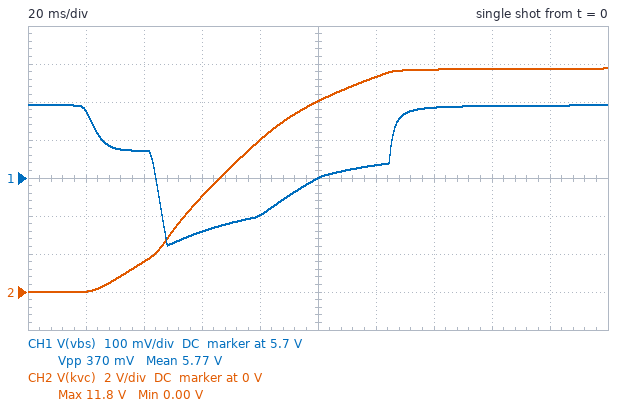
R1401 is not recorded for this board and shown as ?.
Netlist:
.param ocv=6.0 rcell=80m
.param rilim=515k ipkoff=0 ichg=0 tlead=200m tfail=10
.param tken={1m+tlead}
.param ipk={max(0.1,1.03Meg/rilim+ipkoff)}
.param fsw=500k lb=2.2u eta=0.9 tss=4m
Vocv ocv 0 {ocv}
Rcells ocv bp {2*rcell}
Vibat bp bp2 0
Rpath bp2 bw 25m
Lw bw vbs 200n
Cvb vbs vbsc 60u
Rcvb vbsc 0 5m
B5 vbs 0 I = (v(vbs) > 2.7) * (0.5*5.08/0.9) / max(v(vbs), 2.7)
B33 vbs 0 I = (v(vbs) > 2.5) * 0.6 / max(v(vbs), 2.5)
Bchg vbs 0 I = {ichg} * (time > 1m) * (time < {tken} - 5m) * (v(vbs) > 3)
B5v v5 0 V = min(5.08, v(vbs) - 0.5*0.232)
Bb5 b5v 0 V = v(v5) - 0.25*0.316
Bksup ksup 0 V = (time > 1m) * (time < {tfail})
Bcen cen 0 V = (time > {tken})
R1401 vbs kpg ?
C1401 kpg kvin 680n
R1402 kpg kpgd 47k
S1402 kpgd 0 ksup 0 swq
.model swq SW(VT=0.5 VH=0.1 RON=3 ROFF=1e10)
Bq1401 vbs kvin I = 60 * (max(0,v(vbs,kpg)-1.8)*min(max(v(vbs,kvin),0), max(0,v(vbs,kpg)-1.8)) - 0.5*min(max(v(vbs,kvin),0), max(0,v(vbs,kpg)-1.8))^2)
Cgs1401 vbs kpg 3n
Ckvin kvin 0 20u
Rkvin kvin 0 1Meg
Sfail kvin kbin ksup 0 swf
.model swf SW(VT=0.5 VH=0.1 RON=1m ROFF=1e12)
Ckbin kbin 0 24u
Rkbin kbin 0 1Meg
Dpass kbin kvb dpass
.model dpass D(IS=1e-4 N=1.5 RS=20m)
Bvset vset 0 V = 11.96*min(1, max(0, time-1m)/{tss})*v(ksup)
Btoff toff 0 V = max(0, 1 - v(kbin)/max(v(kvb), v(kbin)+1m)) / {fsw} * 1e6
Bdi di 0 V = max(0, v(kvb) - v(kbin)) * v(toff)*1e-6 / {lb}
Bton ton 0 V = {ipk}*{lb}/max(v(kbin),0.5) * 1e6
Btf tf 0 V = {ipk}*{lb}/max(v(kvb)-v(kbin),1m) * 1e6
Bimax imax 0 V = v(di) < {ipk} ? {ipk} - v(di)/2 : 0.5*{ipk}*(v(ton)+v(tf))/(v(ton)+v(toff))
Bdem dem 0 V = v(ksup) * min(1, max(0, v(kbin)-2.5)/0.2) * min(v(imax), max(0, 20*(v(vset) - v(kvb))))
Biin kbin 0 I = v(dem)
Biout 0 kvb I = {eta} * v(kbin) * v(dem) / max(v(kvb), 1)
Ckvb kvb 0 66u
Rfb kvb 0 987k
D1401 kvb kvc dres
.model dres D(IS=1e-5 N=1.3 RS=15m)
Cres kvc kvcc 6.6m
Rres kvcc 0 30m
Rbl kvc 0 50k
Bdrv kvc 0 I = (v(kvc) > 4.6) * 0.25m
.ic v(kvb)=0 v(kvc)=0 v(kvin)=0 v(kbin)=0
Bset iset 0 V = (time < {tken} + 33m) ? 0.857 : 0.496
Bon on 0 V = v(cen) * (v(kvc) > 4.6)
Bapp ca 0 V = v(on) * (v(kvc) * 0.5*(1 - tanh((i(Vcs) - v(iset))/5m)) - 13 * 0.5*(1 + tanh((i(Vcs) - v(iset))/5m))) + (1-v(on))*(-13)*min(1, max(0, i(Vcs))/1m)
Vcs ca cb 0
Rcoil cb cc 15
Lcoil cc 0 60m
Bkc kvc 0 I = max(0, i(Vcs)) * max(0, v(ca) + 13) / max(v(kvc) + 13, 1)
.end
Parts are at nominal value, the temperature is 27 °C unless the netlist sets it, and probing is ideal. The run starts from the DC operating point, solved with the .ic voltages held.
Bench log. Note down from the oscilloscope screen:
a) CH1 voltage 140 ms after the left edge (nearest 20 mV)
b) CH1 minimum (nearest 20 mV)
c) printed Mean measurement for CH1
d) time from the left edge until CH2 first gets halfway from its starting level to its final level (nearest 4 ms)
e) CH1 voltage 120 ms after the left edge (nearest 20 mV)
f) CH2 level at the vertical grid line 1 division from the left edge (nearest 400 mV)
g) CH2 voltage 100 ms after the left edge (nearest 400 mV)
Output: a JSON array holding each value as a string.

["5.88 V", "5.52 V", "5.77 V", "64 ms", "5.74 V", "0 V", "10.0 V"]
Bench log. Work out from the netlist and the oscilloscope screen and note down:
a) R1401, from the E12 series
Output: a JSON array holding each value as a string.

["120 kΩ"]
